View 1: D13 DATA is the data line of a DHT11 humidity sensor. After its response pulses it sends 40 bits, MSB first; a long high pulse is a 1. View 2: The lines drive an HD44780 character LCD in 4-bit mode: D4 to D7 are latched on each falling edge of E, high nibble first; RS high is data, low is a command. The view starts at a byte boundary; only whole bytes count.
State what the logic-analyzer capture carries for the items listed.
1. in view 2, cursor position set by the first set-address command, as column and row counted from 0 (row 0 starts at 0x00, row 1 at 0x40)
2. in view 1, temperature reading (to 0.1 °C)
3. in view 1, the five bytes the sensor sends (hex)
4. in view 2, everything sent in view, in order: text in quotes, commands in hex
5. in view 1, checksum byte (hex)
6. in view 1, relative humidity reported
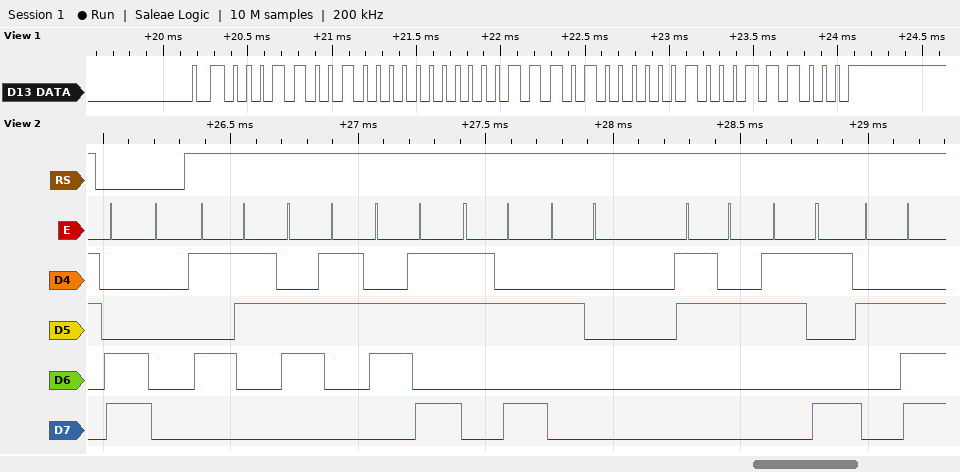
column 0, row 1
29.2 °C
19 00 1D 02 38
0xC0 "Sck: 29."
0x38
25 %
